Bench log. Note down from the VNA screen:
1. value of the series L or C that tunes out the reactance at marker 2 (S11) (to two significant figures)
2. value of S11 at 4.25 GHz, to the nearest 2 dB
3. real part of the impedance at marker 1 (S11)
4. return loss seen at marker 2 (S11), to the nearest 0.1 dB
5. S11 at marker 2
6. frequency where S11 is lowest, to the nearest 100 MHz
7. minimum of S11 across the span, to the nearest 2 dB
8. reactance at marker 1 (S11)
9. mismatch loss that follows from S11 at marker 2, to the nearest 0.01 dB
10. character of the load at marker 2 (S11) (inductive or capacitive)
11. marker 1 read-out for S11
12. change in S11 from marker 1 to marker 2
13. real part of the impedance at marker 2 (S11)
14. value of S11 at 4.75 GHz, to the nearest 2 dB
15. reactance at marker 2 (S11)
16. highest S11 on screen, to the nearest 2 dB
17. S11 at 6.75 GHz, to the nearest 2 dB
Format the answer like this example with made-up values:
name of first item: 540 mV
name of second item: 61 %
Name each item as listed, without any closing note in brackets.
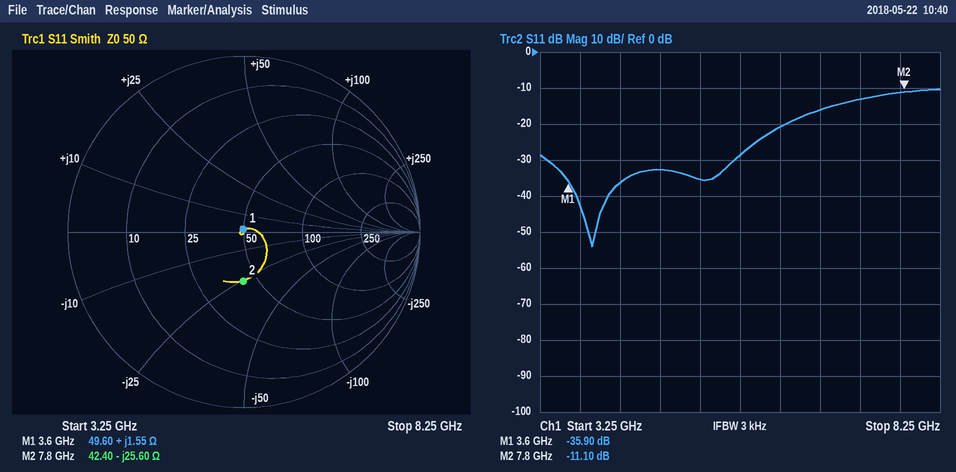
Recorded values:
value of the series L or C that tunes out the reactance at marker 2 (S11): 520 pH
value of S11 at 4.25 GHz, to the nearest 2 dB: -36 dB
real part of the impedance at marker 1: 49.60 Ω
return loss seen at marker 2 (S11), to the nearest 0.1 dB: 11.1 dB
S11 at marker 2: -11.10 dB
frequency where S11 is lowest, to the nearest 100 MHz: 3.9 GHz
minimum of S11 across the span, to the nearest 2 dB: -54 dB
reactance at marker 1: +1.55 Ω
mismatch loss that follows from S11 at marker 2, to the nearest 0.01 dB: 0.35 dB
character of the load at marker 2 (S11): capacitive
marker 1 read-out for S11: -35.90 dB
change in S11 from marker 1 to marker 2: 24.80 dB
real part of the impedance at marker 2: 42.40 Ω
value of S11 at 4.75 GHz, to the nearest 2 dB: -32 dB
reactance at marker 2: -25.60 Ω
highest S11 on screen, to the nearest 2 dB: -10 dB
S11 at 6.75 GHz, to the nearest 2 dB: -16 dB
